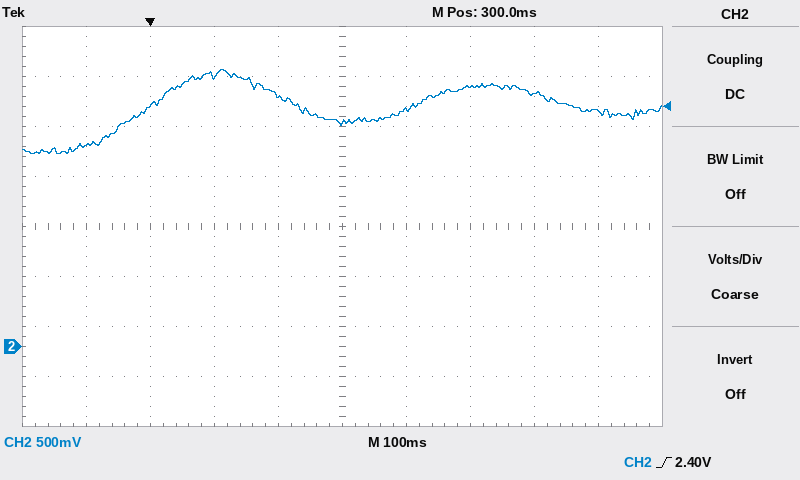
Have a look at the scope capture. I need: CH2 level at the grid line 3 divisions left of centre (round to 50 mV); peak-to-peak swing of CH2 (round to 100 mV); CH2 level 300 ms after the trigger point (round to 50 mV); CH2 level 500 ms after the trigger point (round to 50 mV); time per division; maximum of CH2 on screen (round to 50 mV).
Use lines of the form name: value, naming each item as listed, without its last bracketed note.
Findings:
CH2 level at the grid line 3 divisions left of centre: 2.40 V
peak-to-peak swing of CH2: 800 mV
CH2 level 300 ms after the trigger point: 2.25 V
CH2 level 500 ms after the trigger point: 2.60 V
time per division: 100 ms
maximum of CH2 on screen: 2.75 V
